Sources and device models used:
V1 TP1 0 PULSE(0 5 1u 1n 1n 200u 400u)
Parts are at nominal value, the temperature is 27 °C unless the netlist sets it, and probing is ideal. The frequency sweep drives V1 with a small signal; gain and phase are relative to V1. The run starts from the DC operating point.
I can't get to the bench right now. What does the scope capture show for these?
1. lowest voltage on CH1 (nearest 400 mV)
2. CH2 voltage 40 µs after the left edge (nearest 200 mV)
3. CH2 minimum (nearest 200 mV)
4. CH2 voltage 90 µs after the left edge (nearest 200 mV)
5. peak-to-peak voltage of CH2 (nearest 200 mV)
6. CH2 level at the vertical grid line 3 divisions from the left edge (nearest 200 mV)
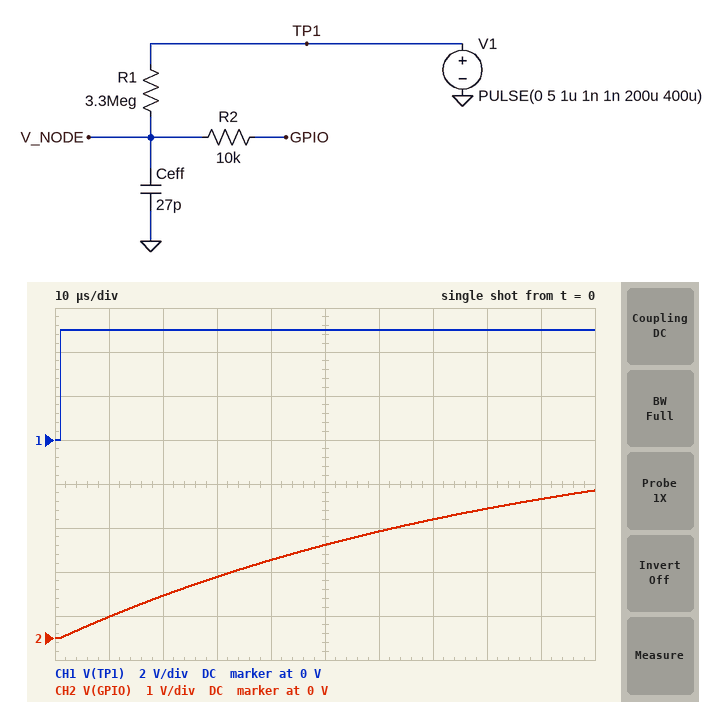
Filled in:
0 V
1.8 V
0 V
3.2 V
3.4 V
1.4 V
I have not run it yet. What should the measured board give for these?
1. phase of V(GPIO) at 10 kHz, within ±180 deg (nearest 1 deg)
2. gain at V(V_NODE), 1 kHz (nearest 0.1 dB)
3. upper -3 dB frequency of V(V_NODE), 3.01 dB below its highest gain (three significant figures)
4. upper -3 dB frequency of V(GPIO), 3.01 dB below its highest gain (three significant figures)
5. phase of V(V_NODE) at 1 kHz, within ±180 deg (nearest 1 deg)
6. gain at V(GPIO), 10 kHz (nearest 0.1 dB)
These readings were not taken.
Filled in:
-80 deg
-1.2 dB
1.79 kHz
1.79 kHz
-29 deg
-15.1 dB
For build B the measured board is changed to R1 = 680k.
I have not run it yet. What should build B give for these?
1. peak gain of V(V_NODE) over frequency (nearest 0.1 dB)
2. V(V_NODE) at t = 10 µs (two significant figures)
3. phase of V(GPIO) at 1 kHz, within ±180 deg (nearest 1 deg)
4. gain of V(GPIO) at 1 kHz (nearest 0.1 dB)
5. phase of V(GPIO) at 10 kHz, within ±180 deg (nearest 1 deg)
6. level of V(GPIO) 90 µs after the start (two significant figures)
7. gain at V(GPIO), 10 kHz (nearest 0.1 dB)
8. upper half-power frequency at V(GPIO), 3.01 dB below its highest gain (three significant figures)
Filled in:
0 dB
1.9 V
-7 deg
-0.1 dB
-49 deg
5.0 V
-3.7 dB
8.67 kHz
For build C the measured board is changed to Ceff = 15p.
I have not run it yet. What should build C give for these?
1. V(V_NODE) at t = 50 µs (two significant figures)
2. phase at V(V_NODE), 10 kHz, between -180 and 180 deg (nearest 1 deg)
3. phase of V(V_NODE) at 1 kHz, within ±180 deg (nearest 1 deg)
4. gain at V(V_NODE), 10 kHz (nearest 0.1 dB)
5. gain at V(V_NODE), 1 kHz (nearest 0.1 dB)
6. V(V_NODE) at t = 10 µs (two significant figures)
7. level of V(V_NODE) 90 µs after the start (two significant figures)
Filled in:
3.1 V
-72 deg
-17 deg
-10.3 dB
-0.4 dB
830 mV
4.2 V
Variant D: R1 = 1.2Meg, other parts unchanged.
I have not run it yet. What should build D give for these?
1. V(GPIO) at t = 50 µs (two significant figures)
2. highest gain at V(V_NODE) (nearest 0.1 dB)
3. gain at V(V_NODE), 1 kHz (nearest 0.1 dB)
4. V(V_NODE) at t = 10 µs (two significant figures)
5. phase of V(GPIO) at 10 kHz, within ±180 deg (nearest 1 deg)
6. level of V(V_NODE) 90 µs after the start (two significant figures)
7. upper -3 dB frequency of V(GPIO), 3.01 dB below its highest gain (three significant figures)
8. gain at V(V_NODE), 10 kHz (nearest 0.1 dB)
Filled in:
3.9 V
0 dB
-0.2 dB
1.2 V
-64 deg
4.7 V
4.91 kHz
-7.1 dB
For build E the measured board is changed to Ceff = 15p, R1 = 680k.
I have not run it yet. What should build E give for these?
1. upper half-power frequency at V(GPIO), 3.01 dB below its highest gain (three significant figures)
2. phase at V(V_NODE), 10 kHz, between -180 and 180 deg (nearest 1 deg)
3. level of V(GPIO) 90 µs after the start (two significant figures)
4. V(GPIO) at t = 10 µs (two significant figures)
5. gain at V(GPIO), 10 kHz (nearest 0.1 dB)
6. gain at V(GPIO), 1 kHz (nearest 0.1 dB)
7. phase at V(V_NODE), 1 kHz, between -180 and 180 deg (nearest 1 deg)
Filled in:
15.6 kHz
-33 deg
5.0 V
2.9 V
-1.5 dB
0 dB
-4 deg
